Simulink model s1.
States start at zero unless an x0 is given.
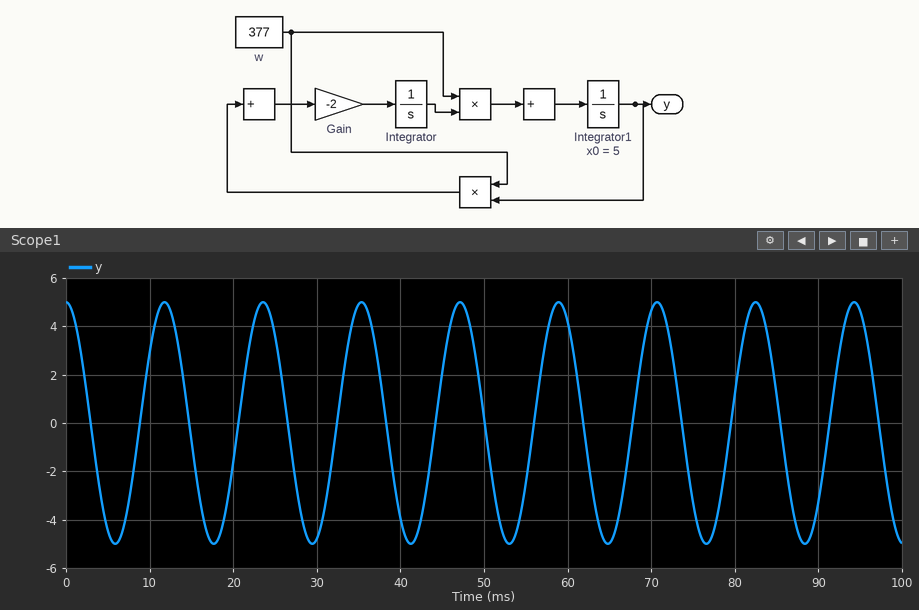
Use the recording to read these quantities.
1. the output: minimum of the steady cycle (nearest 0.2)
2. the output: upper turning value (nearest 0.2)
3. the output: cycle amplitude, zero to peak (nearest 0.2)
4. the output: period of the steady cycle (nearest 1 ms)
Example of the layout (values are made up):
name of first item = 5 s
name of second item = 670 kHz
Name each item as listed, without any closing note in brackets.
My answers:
the output: minimum of the steady cycle = -5.0
the output: upper turning value = 5.0
the output: cycle amplitude, zero to peak = 5.0
the output: period of the steady cycle = 12 ms
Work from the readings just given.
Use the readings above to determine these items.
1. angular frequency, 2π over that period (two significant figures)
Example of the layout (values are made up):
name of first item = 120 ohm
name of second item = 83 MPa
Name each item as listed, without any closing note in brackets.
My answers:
angular frequency, 2π over that period = 0.52 rad/ms
